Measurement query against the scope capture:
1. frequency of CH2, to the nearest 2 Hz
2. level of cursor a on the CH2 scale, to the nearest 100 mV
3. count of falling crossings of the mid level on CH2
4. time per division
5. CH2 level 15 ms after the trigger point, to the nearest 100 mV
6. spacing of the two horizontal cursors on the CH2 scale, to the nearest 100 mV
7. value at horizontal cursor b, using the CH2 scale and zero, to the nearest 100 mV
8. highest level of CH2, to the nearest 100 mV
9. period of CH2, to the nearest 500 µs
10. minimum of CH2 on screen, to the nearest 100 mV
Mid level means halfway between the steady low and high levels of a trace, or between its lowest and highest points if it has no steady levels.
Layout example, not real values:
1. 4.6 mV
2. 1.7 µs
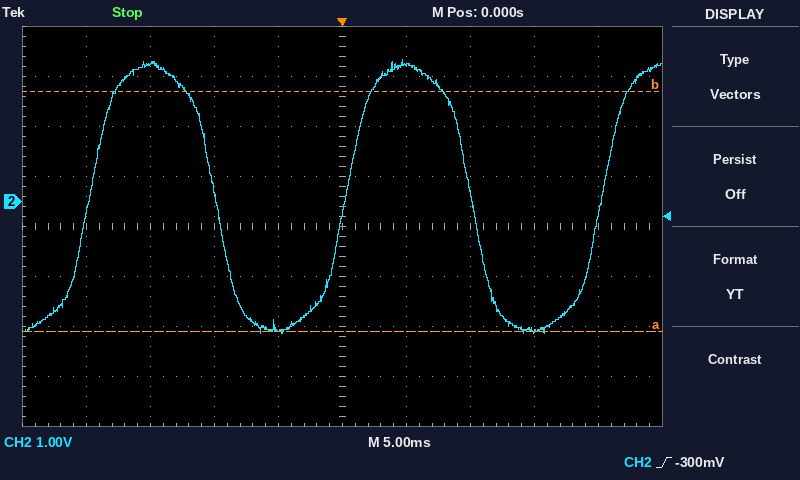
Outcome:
1. 50 Hz
2. -2.6 V
3. 2
4. 5 ms
5. -2.6 V
6. 4.8 V
7. 2.2 V
8. 2.8 V
9. 20.0 ms
10. -2.6 V
